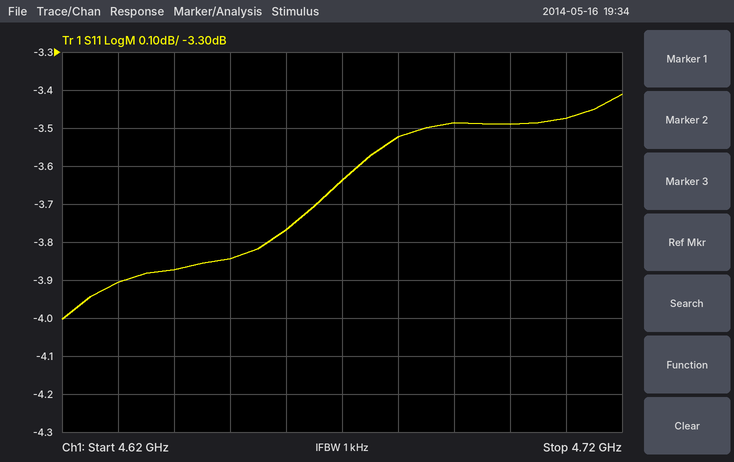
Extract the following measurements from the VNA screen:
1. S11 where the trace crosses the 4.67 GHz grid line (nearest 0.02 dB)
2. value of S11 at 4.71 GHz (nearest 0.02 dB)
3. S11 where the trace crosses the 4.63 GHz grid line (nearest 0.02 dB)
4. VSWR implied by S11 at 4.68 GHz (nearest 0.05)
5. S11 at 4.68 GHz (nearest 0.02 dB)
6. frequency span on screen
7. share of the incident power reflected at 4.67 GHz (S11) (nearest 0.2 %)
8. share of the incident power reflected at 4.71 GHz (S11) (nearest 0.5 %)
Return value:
-3.64 dB
-3.48 dB
-3.90 dB
5.00
-3.52 dB
100 MHz
43.2 %
45.0 %
